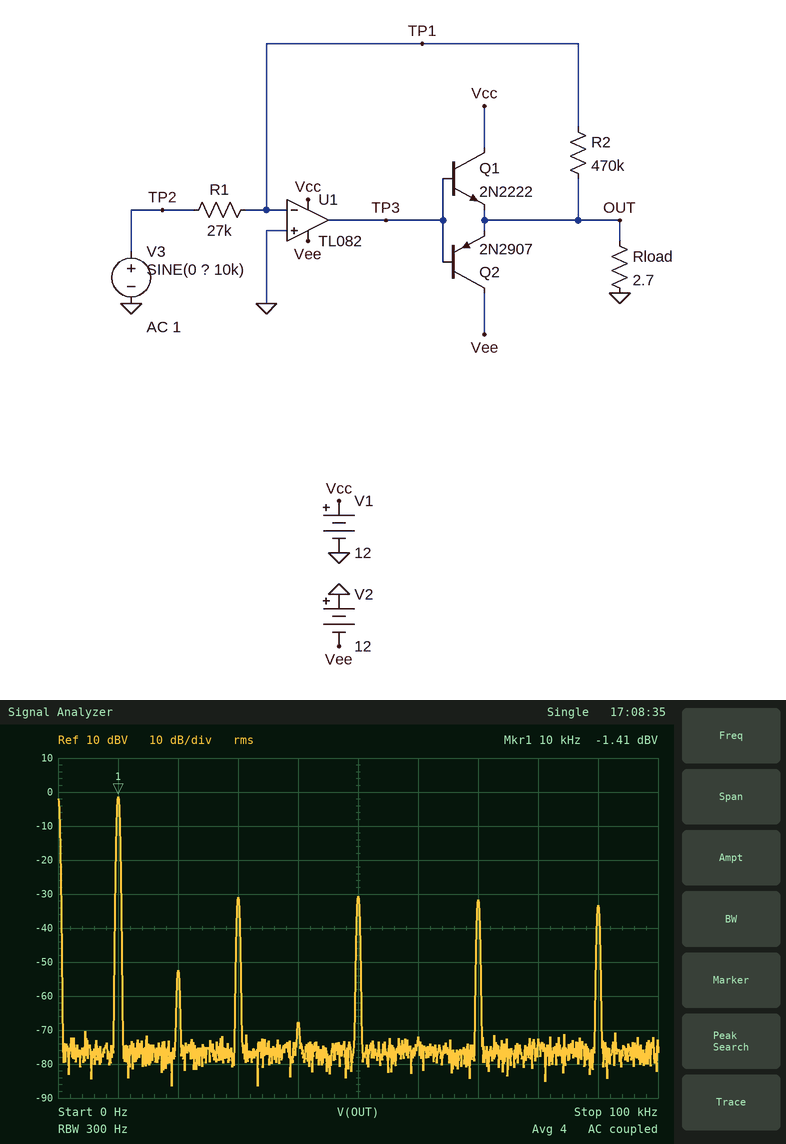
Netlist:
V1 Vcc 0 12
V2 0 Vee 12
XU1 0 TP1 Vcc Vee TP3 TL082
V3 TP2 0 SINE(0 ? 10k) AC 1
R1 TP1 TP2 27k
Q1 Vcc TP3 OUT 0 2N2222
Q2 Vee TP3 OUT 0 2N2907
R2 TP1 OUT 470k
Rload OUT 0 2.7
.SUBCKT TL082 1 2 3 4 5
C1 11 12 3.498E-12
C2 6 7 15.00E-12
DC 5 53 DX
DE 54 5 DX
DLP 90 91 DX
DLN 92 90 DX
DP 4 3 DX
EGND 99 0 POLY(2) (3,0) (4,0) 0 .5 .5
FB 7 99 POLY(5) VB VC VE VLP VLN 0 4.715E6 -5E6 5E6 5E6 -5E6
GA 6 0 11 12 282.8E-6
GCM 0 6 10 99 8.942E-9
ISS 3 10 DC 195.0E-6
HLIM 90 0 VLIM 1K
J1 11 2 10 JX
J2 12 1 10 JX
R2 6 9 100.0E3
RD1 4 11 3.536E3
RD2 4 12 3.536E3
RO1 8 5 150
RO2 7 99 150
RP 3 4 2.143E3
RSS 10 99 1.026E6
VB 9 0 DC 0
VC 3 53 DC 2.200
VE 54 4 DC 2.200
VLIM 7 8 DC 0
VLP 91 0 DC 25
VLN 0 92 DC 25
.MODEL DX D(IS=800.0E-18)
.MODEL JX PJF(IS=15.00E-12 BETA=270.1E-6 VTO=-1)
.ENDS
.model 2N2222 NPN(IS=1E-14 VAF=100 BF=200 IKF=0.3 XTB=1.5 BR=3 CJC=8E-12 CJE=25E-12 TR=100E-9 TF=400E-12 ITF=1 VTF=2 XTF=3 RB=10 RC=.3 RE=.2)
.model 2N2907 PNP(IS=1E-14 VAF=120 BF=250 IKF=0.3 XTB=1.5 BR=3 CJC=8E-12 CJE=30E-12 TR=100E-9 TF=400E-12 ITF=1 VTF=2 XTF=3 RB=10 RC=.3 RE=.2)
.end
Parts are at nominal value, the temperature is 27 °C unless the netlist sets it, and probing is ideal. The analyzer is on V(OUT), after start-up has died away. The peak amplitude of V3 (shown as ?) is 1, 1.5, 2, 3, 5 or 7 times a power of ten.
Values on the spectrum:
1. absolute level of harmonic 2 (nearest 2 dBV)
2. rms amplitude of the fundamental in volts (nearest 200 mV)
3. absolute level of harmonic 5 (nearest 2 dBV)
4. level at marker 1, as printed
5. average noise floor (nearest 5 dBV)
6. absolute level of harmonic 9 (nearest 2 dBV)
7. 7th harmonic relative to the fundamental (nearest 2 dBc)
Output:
-52 dBV
800 mV
-30 dBV
-1.41 dBV
-75 dBV
-34 dBV
-30 dBc
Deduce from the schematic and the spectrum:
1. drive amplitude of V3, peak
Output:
70 mV
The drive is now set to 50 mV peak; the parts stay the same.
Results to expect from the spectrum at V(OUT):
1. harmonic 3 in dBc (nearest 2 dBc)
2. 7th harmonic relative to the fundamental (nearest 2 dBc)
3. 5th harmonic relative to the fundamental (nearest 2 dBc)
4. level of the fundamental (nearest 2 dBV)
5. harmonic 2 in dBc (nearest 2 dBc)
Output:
-26 dBc
-28 dBc
-26 dBc
-4 dBV
-52 dBc
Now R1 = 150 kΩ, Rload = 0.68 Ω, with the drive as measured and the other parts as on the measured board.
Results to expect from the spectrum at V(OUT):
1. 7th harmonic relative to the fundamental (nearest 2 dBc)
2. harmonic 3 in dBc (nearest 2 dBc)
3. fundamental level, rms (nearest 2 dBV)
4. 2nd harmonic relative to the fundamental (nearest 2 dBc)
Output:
-28 dBc
-26 dBc
-16 dBV
-54 dBc
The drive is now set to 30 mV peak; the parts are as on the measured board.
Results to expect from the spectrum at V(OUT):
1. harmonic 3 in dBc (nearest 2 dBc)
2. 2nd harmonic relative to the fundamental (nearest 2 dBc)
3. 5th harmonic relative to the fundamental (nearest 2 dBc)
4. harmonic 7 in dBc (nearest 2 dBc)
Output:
-22 dBc
-54 dBc
-22 dBc
-26 dBc
